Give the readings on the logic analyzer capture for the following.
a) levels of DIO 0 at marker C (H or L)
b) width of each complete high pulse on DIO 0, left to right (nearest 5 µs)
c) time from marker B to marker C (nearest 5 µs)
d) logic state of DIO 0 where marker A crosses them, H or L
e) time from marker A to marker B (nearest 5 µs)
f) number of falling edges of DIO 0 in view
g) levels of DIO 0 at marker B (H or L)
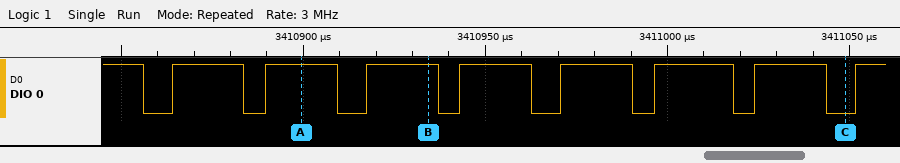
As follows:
DIO 0=L
20 µs, 20 µs, 20 µs, 20 µs, 20 µs, 20 µs, 20 µs
115 µs
DIO 0=H
35 µs
8
DIO 0=H
